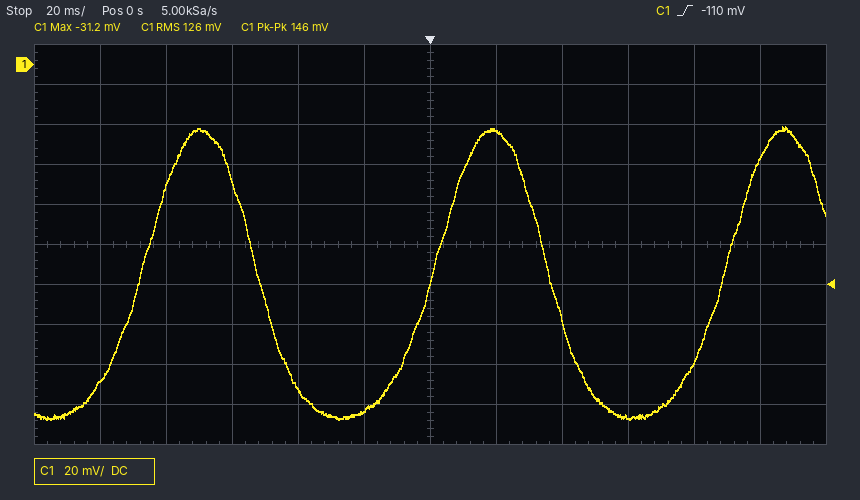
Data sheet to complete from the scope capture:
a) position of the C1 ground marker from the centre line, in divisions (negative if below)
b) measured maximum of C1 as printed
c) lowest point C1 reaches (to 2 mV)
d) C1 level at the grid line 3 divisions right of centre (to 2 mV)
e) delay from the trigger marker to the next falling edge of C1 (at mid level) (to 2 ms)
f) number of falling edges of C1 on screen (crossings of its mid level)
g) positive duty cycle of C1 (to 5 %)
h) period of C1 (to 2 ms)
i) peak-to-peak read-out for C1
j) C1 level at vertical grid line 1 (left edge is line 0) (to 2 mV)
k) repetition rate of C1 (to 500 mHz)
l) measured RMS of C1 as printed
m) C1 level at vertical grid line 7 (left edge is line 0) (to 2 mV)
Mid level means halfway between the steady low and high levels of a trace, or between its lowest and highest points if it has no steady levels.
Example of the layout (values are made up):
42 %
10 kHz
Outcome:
+4.5 div
-31.2 mV
-178 mV
-176 mV
36 ms
2
40 %
88 ms
146 mV
-158 mV
11.5 Hz
126 mV
-34 mV
